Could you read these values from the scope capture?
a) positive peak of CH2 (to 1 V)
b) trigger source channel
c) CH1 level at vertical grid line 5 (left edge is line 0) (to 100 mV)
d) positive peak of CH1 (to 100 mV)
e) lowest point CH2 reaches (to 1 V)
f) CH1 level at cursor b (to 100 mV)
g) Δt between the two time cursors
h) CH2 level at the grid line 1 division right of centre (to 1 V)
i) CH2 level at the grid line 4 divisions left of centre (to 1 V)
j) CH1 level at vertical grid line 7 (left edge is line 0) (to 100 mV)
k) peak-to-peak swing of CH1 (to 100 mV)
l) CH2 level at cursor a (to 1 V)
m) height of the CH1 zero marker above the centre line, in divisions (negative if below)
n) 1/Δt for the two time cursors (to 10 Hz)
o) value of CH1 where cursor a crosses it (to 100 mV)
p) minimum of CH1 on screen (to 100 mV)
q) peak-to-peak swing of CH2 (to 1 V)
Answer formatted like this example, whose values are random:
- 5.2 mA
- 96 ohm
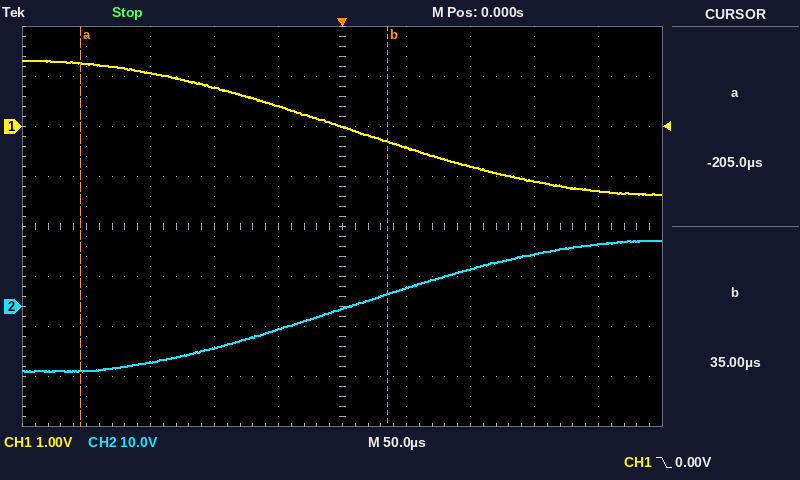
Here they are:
- 13 V
- CH1
- 0.0 V
- 1.3 V
- -13 V
- -300 mV
- 240 µs
- 4 V
- -13 V
- -800 mV
- 2.7 V
- -13 V
- +2.0 div
- 4.17 kHz
- 1.3 V
- -1.4 V
- 26 V
